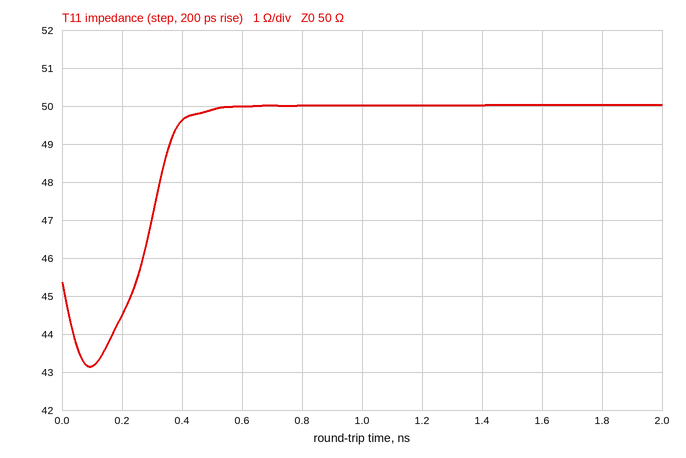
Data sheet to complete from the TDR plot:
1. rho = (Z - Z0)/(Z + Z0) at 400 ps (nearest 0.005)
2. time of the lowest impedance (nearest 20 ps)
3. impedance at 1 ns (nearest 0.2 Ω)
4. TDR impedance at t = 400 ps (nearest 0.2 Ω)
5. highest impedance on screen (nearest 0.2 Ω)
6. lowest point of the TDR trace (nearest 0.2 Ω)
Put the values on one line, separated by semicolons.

-0.005; 100 ps; 50.0 Ω; 49.6 Ω; 50.0 Ω; 43.2 Ω
